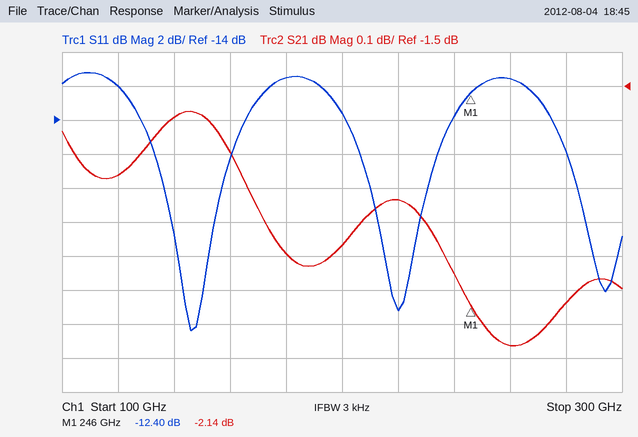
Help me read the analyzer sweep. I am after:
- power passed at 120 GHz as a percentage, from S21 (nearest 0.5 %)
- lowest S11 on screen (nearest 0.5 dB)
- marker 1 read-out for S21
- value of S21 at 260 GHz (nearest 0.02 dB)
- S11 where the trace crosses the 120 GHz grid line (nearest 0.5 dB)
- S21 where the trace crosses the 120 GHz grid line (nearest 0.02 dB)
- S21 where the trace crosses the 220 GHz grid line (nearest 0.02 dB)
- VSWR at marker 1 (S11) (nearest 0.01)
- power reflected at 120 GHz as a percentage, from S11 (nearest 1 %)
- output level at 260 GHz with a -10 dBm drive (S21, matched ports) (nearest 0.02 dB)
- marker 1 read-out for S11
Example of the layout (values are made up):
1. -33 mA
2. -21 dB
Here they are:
1. 66.5 %
2. -26.5 dB
3. -2.14 dB
4. -2.26 dB
5. -12.0 dB
6. -1.76 dB
7. -1.84 dB
8. 1.63
9. 6 %
10. -12.26 dBm
11. -12.40 dB
